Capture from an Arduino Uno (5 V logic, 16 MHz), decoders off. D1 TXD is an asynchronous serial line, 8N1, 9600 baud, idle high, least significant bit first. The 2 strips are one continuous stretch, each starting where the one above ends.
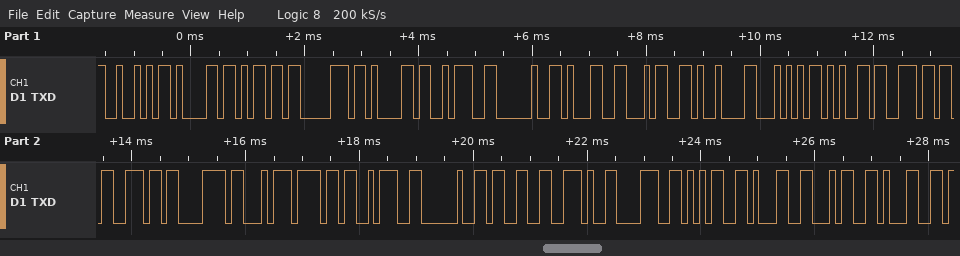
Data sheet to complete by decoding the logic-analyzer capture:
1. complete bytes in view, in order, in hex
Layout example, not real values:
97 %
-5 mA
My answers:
52 61 6D 70 61 3A 20 31 34 09 54 65 6E 73 C3 A3 6F 3A 20 33 2E 38 35 31 34 31
